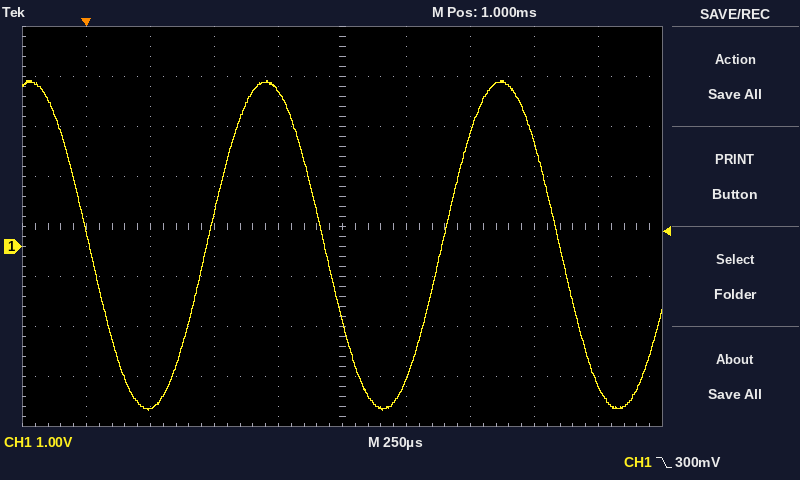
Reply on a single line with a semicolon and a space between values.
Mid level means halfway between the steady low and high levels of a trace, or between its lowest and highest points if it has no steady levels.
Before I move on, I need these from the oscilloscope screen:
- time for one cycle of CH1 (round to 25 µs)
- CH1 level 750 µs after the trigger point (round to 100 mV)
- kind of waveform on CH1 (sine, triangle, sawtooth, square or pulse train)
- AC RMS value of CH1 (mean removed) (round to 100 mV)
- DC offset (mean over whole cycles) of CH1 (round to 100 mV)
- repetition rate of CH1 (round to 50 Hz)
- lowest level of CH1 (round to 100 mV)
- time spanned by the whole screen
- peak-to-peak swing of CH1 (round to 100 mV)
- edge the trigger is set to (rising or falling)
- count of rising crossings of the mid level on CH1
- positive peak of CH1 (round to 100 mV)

925 µs; 3.1 V; sine; 2.3 V; 0.0 V; 1.10 kHz; -3.3 V; 2.5 ms; 6.6 V; falling; 2; 3.3 V
